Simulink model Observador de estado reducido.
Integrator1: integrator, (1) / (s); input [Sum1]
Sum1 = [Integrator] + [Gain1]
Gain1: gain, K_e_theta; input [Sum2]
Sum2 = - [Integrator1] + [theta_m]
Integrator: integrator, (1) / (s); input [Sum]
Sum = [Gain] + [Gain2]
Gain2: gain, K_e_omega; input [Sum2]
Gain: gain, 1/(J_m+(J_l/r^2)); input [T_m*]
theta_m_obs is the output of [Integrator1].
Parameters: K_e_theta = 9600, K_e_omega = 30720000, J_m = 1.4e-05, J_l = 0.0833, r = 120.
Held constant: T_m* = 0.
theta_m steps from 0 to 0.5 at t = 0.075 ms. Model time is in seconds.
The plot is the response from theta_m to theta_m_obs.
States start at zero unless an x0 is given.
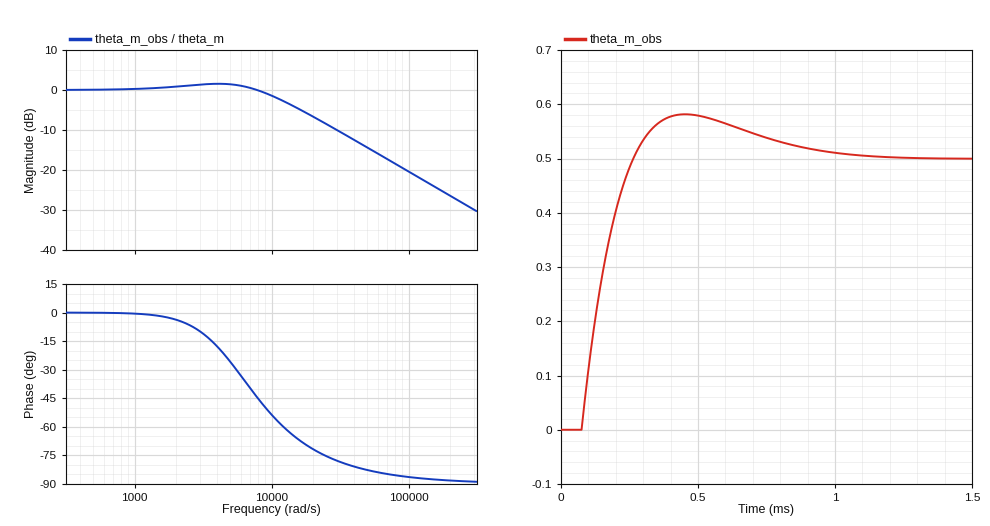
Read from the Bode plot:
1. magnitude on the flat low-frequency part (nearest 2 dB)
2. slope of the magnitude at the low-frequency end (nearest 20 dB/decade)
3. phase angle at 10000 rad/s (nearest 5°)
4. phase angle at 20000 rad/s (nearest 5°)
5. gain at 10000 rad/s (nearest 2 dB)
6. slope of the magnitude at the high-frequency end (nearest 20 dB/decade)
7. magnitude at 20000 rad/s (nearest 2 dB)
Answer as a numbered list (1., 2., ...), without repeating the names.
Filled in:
1. 0 dB
2. 0 dB/decade
3. -55°
4. -70°
5. -2 dB
6. -20 dB/decade
7. -6 dB
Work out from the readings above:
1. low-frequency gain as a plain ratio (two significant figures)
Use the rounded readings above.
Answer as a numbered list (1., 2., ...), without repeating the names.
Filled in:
1. 1.0
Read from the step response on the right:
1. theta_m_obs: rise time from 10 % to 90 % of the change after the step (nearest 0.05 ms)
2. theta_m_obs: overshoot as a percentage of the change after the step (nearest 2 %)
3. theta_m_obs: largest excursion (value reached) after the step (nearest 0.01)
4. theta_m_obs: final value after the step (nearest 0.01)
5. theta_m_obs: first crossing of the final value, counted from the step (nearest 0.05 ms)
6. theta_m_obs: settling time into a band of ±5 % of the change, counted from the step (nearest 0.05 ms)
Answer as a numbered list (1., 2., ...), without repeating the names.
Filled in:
1. 0.15 ms
2. 16 %
3. 0.58
4. 0.50
5. 0.20 ms
6. 0.75 ms
